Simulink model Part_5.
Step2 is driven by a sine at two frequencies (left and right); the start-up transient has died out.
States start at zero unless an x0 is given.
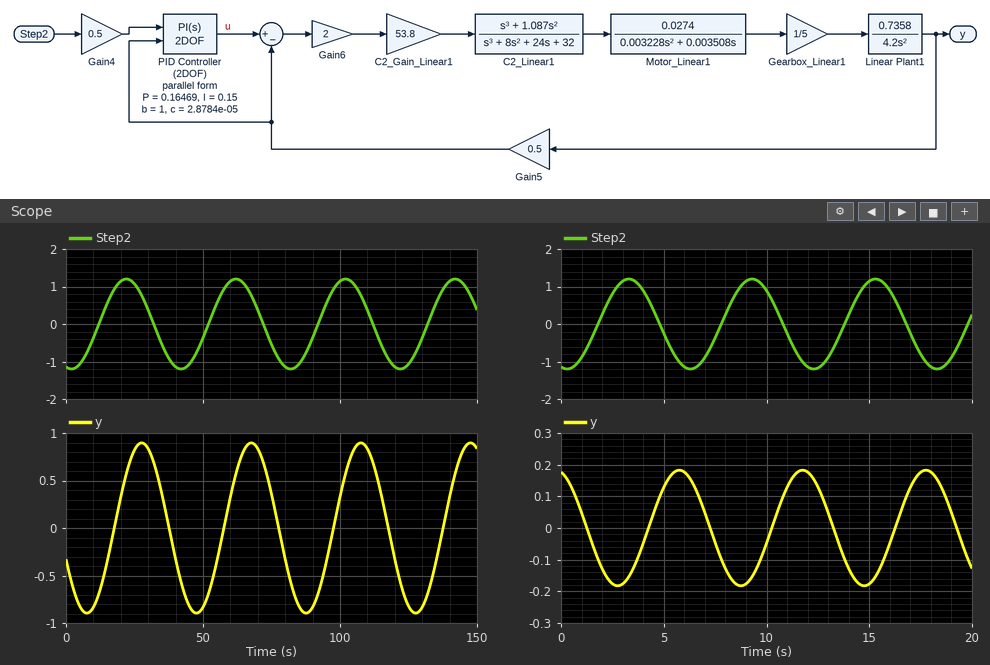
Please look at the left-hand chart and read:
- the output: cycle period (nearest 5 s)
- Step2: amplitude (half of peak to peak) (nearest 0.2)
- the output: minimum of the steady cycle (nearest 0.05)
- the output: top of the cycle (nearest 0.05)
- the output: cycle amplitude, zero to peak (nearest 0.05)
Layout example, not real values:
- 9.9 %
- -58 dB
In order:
- 40 s
- 1.2
- -0.90
- 0.90
- 0.90
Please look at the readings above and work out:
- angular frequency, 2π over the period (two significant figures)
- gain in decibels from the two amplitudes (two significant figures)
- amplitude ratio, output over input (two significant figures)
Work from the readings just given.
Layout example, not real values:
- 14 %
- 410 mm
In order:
- 0.16 rad/s
- -2.5 dB
- 0.75
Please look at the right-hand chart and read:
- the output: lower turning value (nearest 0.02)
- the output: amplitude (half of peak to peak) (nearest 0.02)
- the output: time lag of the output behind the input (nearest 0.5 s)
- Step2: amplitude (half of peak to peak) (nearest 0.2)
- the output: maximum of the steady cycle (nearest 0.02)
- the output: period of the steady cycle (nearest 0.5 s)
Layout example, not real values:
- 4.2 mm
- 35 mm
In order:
- -0.18
- 0.18
- 2.5 s
- 1.2
- 0.18
- 6.0 s
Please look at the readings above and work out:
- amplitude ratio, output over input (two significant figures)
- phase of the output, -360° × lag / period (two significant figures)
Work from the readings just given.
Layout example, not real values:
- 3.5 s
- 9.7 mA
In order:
- 0.15
- -150°
